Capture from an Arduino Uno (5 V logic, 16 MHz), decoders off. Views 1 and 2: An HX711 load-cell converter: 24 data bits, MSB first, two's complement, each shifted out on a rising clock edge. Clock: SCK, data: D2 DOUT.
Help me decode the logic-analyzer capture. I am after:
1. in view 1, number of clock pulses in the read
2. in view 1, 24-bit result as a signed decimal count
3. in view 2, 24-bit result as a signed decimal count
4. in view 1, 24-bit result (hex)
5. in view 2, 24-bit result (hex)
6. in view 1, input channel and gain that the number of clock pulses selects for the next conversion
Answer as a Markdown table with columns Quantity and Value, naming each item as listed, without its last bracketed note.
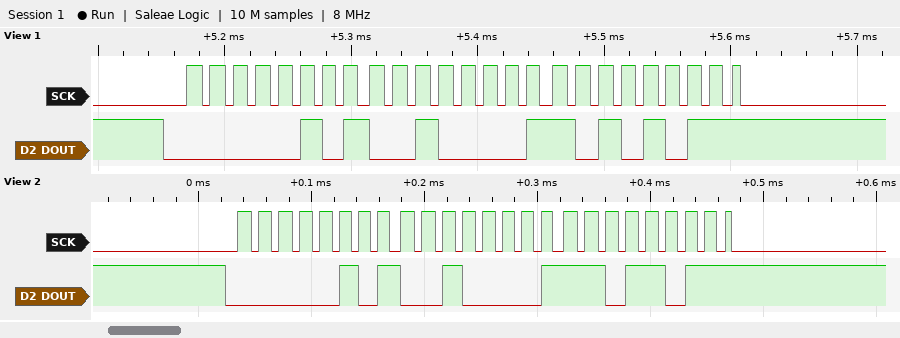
| Quantity | Value |
|---|---|
| in view 1, number of clock pulses in the read | 25 |
| in view 1, 24-bit result as a signed decimal count | 336299 |
| in view 2, 24-bit result as a signed decimal count | 336347 |
| in view 1, 24-bit result | 0x0521AB |
| in view 2, 24-bit result | 0x0521DB |
| in view 1, input channel and gain that the number of clock pulses selects for the next conversion | channel A, gain 128 |
